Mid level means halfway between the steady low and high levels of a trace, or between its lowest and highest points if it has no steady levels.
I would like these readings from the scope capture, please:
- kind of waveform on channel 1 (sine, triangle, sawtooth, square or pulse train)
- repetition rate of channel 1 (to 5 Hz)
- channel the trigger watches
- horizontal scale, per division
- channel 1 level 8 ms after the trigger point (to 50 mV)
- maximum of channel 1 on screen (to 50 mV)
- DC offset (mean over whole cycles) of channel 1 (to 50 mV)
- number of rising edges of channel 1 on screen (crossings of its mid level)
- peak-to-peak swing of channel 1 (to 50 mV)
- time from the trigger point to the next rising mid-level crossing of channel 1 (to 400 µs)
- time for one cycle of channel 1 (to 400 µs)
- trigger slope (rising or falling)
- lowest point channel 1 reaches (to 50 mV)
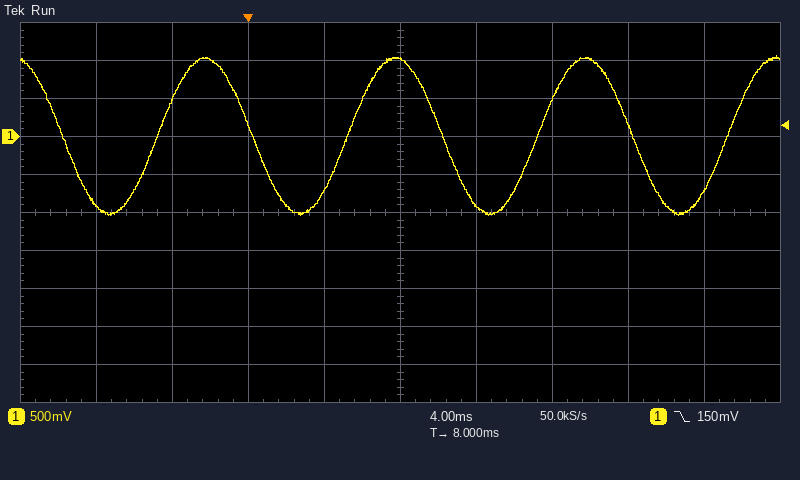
sine
100 Hz
channel 1
4 ms
1.00 V
1.05 V
0 mV
4
2.10 V
5.2 ms
10.0 ms
falling
-1.05 V
